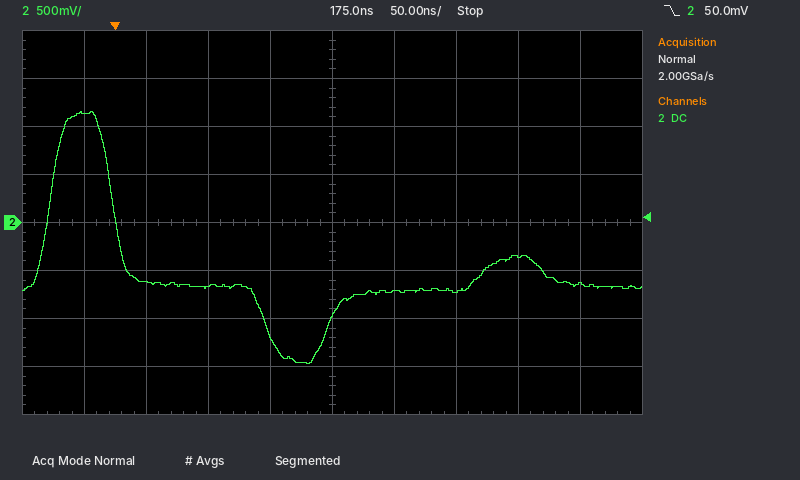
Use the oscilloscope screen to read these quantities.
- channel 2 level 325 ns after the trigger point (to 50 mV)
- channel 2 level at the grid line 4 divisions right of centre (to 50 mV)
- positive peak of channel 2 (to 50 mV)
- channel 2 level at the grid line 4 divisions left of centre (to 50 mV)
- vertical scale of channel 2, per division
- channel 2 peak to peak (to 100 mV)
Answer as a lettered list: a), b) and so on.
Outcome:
a) -350 mV
b) -650 mV
c) 1.15 V
d) 1.15 V
e) 500 mV
f) 2.60 V
